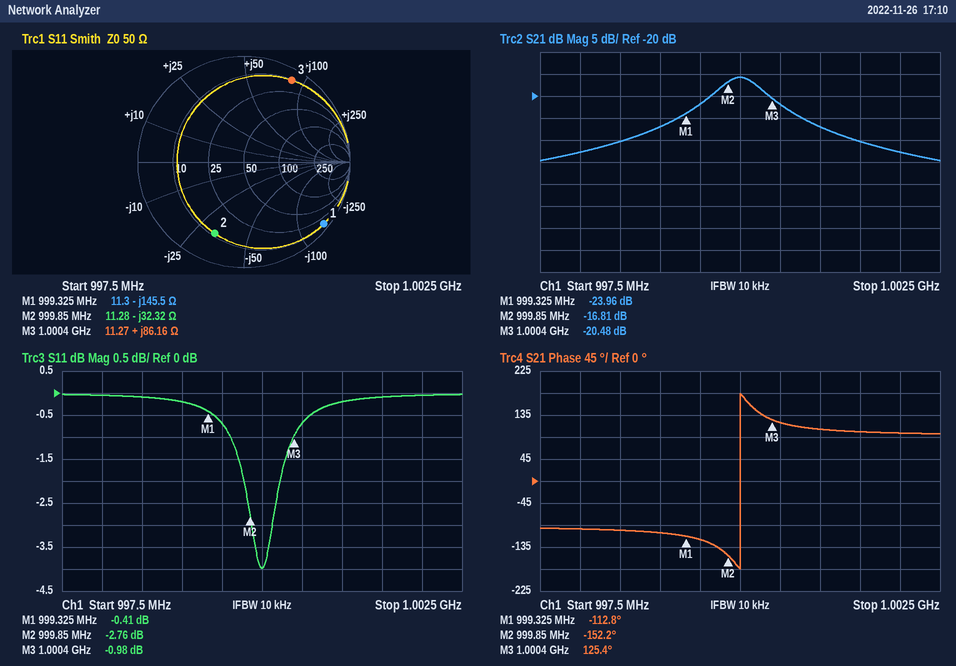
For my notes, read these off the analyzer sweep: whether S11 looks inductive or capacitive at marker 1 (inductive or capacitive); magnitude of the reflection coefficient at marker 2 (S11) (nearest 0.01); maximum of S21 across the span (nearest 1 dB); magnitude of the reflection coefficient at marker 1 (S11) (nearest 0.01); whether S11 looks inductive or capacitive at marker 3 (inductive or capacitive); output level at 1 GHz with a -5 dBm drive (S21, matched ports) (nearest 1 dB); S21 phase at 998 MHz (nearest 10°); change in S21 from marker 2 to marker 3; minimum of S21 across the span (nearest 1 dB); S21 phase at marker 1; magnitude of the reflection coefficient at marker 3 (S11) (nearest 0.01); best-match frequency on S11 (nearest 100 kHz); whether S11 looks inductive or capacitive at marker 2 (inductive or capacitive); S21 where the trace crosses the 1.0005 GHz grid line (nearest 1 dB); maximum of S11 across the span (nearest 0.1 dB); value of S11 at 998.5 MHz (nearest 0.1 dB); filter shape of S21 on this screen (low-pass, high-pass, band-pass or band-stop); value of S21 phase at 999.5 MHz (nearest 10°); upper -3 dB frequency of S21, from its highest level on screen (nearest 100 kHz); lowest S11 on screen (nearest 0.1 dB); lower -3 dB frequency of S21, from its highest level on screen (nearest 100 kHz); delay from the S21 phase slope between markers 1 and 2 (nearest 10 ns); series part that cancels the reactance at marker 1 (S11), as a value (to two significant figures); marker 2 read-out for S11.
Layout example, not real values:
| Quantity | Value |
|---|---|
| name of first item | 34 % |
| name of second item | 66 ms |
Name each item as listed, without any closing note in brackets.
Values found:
| Quantity | Value |
|---|---|
| whether S11 looks inductive or capacitive at marker 1 | capacitive |
| magnitude of the reflection coefficient at marker 2 (S11) | 0.73 |
| maximum of S21 across the span | -16 dB |
| magnitude of the reflection coefficient at marker 1 (S11) | 0.95 |
| whether S11 looks inductive or capacitive at marker 3 | inductive |
| output level at 1 GHz with a -5 dBm drive (S21, matched ports) | -21 dBm |
| S21 phase at 998 MHz | -100° |
| change in S21 from marker 2 to marker 3 | -3.67 dB |
| minimum of S21 across the span | -35 dB |
| S21 phase at marker 1 | -112.8° |
| magnitude of the reflection coefficient at marker 3 (S11) | 0.89 |
| best-match frequency on S11 | 1.0000 GHz |
| whether S11 looks inductive or capacitive at marker 2 | capacitive |
| S21 where the trace crosses the 1.0005 GHz grid line | -22 dB |
| maximum of S11 across the span | 0.0 dB |
| value of S11 at 998.5 MHz | -0.1 dB |
| filter shape of S21 on this screen | band-pass |
| value of S21 phase at 999.5 MHz | -120° |
| upper -3 dB frequency of S21, from its highest level on screen | 1.0003 GHz |
| lowest S11 on screen | -4.0 dB |
| lower -3 dB frequency of S21, from its highest level on screen | 999.7 MHz |
| delay from the S21 phase slope between markers 1 and 2 | 210 ns |
| series part that cancels the reactance at marker 1 (S11), as a value | 23 nH |
| marker 2 read-out for S11 | -2.76 dB |
